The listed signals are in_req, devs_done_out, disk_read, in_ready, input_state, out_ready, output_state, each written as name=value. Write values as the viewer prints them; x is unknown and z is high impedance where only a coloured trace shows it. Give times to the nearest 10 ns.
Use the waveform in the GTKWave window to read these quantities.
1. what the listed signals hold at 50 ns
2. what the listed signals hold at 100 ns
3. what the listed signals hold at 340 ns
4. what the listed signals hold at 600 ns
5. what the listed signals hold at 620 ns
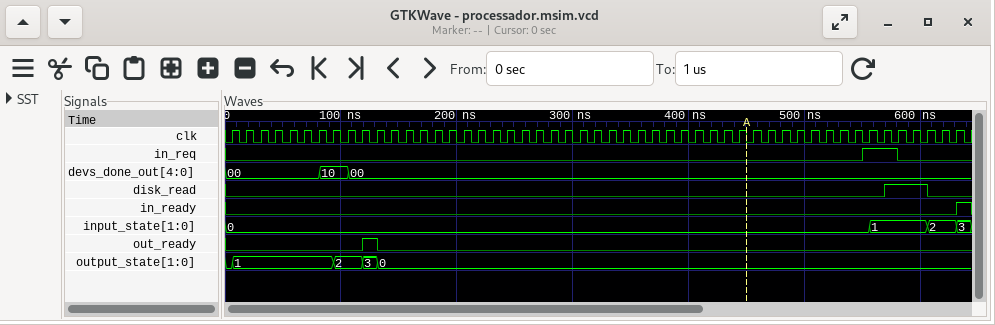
in_req=0, devs_done_out=00, disk_read=0, in_ready=0, input_state=0, out_ready=0, output_state=1
in_req=0, devs_done_out=10, disk_read=0, in_ready=0, input_state=0, out_ready=0, output_state=2
in_req=0, devs_done_out=00, disk_read=0, in_ready=0, input_state=0, out_ready=0, output_state=0
in_req=0, devs_done_out=00, disk_read=1, in_ready=0, input_state=1, out_ready=0, output_state=0
in_req=0, devs_done_out=00, disk_read=0, in_ready=0, input_state=2, out_ready=0, output_state=0
